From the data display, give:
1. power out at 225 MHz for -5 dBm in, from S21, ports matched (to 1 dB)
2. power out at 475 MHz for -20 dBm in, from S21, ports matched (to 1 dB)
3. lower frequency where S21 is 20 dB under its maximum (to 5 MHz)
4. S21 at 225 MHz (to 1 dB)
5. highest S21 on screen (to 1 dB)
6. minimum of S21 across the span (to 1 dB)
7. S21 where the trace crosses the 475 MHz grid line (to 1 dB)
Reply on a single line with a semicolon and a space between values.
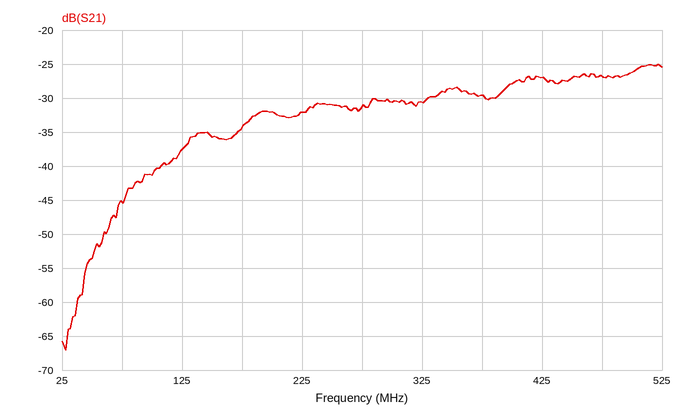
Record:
-37 dBm; -47 dBm; 75 MHz; -32 dB; -25 dB; -67 dB; -27 dB
